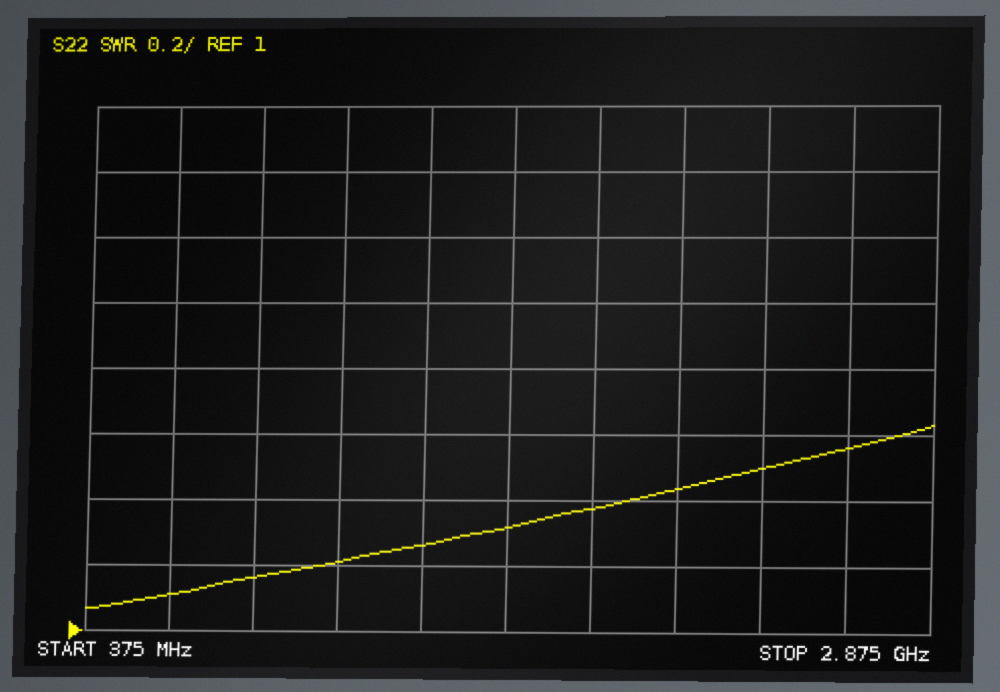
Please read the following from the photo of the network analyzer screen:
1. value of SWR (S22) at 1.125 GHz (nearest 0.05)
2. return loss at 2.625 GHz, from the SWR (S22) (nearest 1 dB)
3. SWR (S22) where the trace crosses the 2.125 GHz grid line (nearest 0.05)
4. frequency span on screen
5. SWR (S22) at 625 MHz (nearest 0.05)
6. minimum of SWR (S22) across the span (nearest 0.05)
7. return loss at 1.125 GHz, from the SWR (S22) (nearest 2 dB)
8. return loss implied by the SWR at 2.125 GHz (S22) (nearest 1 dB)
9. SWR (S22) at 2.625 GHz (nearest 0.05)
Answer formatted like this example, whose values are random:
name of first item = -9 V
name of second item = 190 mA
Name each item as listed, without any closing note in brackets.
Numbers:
value of SWR (S22) at 1.125 GHz = 1.20
return loss at 2.625 GHz, from the SWR (S22) = 13 dB
SWR (S22) where the trace crosses the 2.125 GHz grid line = 1.45
frequency span on screen = 2.5 GHz
SWR (S22) at 625 MHz = 1.10
minimum of SWR (S22) across the span = 1.05
return loss at 1.125 GHz, from the SWR (S22) = 20 dB
return loss implied by the SWR at 2.125 GHz (S22) = 15 dB
SWR (S22) at 2.625 GHz = 1.55
